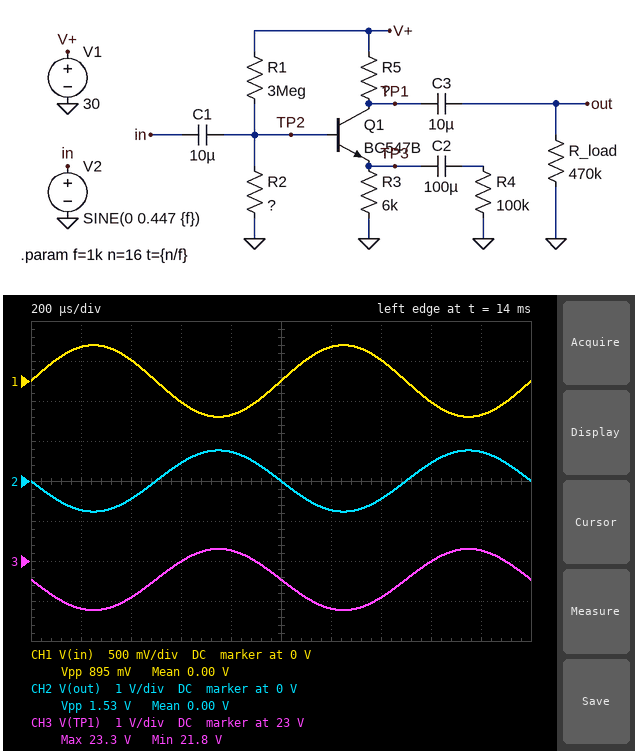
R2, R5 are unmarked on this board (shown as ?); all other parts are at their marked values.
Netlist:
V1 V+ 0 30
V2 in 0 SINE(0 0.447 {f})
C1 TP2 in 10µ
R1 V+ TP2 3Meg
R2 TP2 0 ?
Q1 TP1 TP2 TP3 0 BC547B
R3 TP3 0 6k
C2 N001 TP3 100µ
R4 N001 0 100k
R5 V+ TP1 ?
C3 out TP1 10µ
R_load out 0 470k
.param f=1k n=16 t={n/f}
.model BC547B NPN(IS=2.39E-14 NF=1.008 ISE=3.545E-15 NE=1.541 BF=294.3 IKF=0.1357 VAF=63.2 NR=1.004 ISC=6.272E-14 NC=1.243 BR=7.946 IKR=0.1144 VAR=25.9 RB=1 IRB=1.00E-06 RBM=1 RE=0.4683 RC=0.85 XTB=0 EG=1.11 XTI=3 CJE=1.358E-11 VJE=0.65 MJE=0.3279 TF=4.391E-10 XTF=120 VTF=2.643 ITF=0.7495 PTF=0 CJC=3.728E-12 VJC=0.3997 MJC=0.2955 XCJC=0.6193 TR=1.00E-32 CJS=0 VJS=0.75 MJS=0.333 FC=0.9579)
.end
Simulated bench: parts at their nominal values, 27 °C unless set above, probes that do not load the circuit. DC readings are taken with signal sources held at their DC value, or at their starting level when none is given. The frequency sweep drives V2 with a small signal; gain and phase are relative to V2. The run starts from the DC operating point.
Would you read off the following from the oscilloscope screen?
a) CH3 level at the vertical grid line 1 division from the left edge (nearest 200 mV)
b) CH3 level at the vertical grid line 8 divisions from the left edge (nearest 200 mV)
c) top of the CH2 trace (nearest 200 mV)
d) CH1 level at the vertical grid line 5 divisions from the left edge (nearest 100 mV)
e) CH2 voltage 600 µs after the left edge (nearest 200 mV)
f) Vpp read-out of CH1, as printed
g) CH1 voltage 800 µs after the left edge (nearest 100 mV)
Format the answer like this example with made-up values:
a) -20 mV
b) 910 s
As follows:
a) 21.8 V
b) 23.0 V
c) 800 mV
d) 0 V
e) 400 mV
f) 895 mV
g) -400 mV
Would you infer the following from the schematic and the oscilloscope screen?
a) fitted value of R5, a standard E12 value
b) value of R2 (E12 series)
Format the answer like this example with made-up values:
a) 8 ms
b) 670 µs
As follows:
a) 10 kΩ
b) 820 kΩ
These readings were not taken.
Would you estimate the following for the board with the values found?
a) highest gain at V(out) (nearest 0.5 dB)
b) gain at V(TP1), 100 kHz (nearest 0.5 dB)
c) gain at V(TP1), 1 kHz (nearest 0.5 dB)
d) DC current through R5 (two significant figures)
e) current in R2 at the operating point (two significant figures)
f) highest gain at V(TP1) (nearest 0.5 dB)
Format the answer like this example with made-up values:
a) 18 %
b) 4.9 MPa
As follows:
a) 4.5 dB
b) 4.5 dB
c) 4.5 dB
d) 750 µA
e) 6.2 µA
f) 4.5 dB
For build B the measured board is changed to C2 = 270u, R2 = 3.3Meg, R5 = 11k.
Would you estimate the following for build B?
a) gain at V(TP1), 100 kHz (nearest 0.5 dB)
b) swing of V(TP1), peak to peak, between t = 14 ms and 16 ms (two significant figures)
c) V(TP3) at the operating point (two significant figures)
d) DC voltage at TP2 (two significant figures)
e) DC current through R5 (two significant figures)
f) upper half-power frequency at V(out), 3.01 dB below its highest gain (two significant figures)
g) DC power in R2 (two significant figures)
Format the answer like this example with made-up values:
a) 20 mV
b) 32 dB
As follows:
a) 5.5 dB
b) 1.7 V
c) 8.2 V
d) 8.8 V
e) 1.4 mA
f) 17 MHz
g) 24 µW
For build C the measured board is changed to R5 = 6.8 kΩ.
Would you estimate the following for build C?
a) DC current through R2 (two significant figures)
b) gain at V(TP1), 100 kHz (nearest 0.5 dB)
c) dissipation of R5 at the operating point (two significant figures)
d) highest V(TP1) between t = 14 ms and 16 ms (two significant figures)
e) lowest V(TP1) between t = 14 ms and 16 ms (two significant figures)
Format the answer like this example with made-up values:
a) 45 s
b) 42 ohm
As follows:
a) 6.3 µA
b) 1.5 dB
c) 3.8 mW
d) 25 V
e) 24 V
